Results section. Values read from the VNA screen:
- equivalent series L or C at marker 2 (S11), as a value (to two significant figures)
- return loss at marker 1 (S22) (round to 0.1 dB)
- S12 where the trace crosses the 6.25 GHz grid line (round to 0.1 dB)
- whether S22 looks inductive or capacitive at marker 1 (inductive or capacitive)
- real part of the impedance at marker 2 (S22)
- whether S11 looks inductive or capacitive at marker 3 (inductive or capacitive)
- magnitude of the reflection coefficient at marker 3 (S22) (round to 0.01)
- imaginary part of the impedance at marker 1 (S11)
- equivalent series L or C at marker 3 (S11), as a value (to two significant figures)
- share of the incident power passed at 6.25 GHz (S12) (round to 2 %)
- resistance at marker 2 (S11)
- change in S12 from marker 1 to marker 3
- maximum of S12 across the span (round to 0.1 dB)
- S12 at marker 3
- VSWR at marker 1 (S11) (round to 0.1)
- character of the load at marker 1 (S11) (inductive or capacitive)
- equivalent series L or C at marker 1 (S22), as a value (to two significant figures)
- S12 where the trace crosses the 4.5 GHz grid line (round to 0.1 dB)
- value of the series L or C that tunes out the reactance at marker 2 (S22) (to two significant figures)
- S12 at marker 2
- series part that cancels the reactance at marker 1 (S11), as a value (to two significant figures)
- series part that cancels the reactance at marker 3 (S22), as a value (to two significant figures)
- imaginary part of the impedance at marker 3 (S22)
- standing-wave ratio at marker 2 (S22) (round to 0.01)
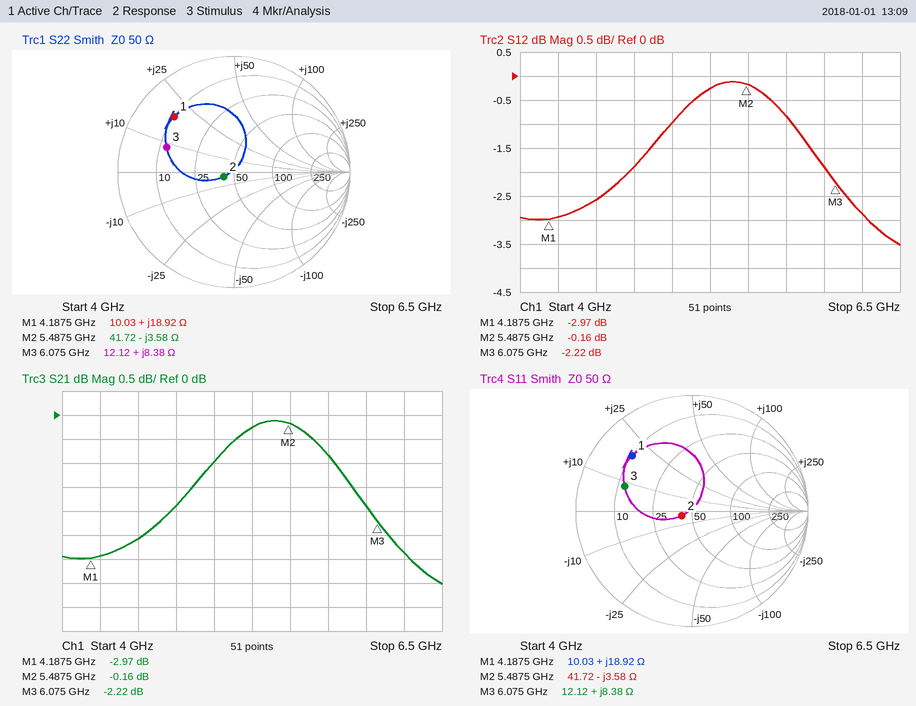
8.1 pF
3.1 dB
-2.9 dB
inductive
41.72 Ω
inductive
0.62
+18.92 Ω
220 pH
52 %
41.72 Ω
0.75 dB
-0.1 dB
-2.22 dB
5.7
inductive
720 pH
-2.6 dB
100 pH
-0.16 dB
2.0 pF
3.1 pF
+8.38 Ω
1.22
